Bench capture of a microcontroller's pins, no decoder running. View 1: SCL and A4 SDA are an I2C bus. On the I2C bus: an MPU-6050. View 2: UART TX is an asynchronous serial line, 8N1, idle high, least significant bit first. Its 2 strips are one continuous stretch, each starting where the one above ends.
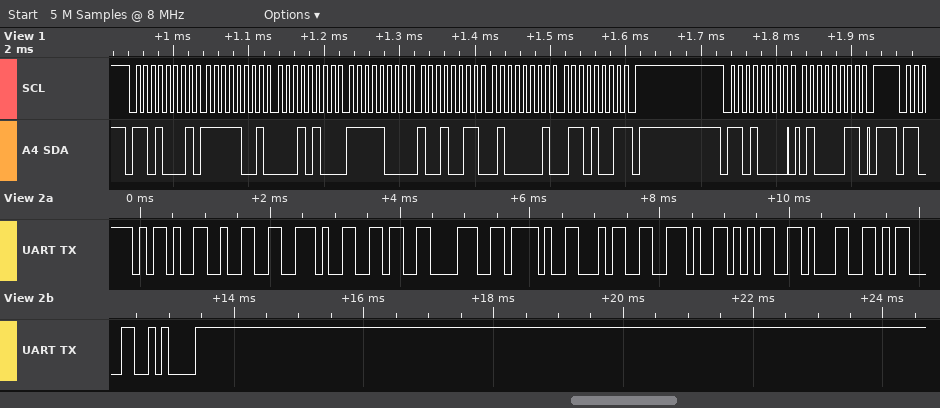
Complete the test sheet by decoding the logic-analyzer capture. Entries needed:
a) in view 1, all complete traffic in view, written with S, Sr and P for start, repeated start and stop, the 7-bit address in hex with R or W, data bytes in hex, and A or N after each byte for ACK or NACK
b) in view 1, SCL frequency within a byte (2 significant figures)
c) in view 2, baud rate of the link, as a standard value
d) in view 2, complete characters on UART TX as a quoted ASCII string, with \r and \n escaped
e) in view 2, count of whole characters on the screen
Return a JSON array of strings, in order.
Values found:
["S 68R A F9 A 14 A F8 A 93 A 41 A 69 N P S 68W A 43 A P", "100 kHz", "9600 baud", "\"-2.68/4.51\\r\\n\"", "12"]
